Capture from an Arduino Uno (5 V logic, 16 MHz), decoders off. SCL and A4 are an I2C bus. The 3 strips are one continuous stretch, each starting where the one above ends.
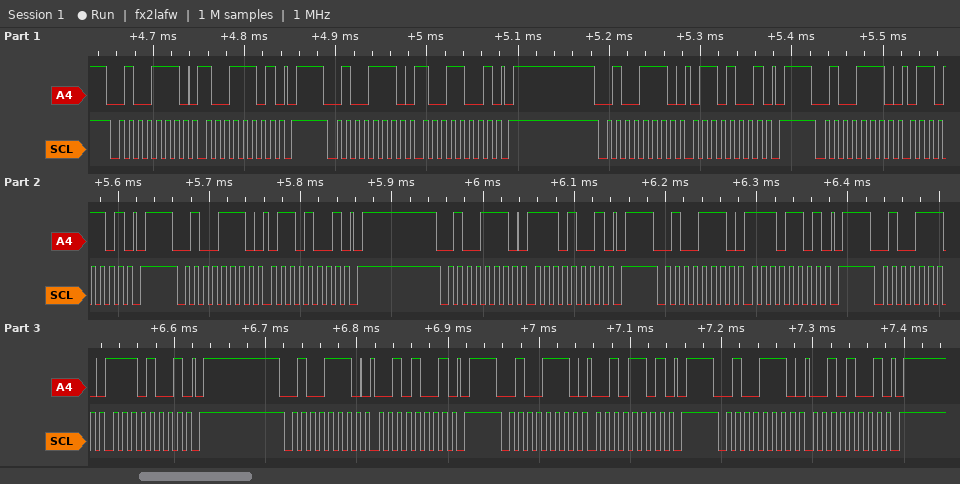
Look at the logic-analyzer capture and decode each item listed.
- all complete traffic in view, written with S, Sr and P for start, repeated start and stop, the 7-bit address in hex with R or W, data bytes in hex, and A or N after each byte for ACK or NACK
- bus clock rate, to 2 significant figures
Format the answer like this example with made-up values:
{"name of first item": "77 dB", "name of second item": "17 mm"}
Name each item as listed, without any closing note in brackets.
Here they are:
{"all complete traffic in view, written with S, Sr and P for start, repeated start and stop, the 7-bit address in hex with R or W, data bytes in hex, and A or N after each byte for ACK or NACK": "S 27W A 9D A P S 27W A 99 A P S 27W A 69 A P S 27W A 6D A P S 27W A 69 A P S 27W A E9 A P S 27W A ED A P S 27W A E9 A P S 27W A 29 A P S 27W A 2D A P S 27W A 29 A P", "bus clock rate, to 2 significant figures": "100 kHz"}
